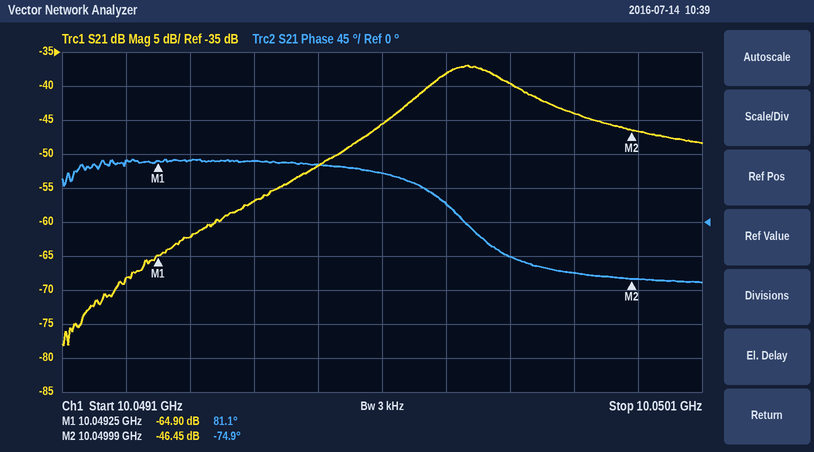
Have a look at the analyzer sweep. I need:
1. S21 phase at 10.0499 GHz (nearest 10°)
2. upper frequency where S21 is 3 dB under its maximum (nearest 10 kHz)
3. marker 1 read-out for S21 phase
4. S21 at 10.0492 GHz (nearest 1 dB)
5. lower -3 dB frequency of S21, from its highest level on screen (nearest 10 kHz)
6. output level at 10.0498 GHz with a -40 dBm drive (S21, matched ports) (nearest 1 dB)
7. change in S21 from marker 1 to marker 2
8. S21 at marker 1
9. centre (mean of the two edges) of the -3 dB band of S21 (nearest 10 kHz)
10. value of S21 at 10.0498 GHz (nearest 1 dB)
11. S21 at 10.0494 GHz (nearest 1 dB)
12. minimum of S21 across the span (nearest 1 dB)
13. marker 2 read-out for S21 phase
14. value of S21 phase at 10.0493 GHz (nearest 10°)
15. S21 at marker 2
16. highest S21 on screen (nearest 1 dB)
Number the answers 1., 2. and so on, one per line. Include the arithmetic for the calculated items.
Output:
1. -70°
2. 10.04981 GHz
3. 81.1°
4. -68 dB
5. 10.04967 GHz
6. -40 dBm + (-40 dB) = -80 dBm
7. -46.45 − (-64.9) = 18.45 dB
8. -64.90 dB
9. 10.04974 GHz
10. -40 dB
11. -57 dB
12. -78 dB
13. -74.9°
14. 80°
15. -46.45 dB
16. -37 dB
